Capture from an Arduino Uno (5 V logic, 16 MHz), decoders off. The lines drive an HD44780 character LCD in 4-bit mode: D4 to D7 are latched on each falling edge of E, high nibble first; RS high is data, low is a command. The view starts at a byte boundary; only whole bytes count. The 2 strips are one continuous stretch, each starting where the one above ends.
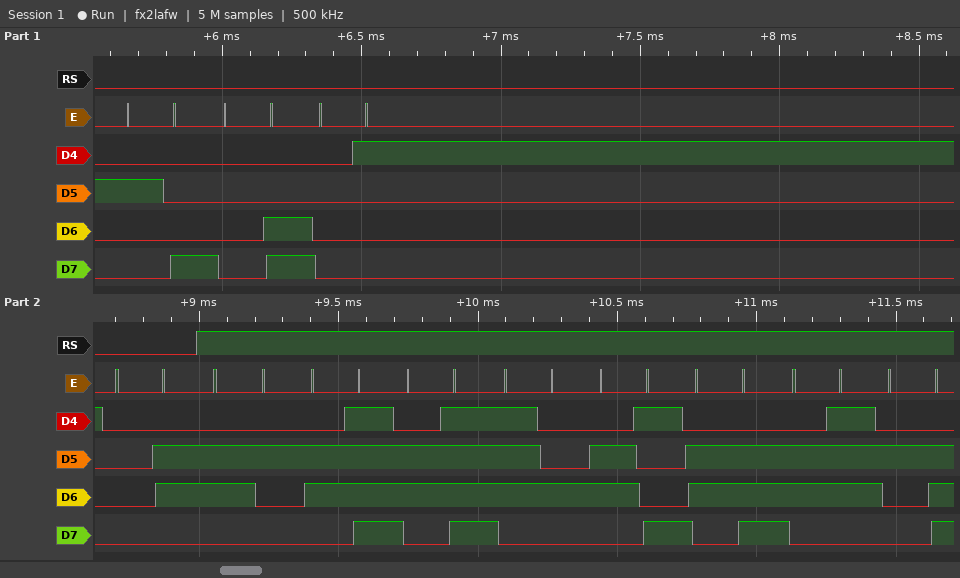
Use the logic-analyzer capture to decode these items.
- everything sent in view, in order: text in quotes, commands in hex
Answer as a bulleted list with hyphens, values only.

- 0x28 0x0C 0x01 0x06 "booting."
